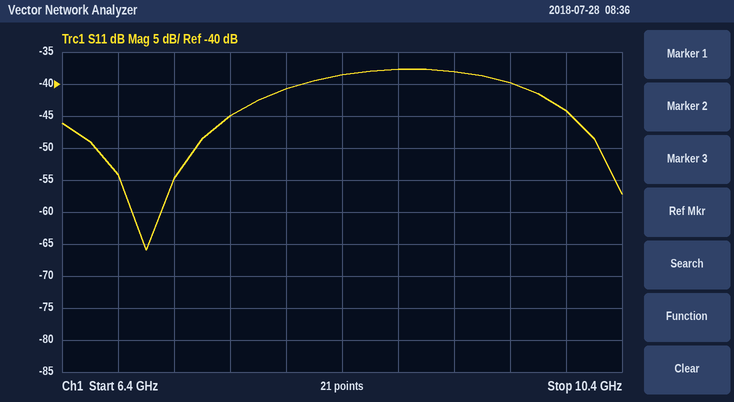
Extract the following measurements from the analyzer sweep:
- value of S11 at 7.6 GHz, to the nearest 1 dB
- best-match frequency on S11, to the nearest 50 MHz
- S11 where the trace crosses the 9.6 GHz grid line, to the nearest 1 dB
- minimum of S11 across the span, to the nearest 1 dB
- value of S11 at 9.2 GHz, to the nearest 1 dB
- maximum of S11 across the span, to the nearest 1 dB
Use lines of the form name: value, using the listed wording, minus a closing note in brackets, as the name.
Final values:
value of S11 at 7.6 GHz, to the nearest 1 dB: -45 dB
best-match frequency on S11, to the nearest 50 MHz: 7.00 GHz
S11 where the trace crosses the 9.6 GHz grid line, to the nearest 1 dB: -40 dB
minimum of S11 across the span, to the nearest 1 dB: -66 dB
value of S11 at 9.2 GHz, to the nearest 1 dB: -38 dB
maximum of S11 across the span, to the nearest 1 dB: -38 dB
